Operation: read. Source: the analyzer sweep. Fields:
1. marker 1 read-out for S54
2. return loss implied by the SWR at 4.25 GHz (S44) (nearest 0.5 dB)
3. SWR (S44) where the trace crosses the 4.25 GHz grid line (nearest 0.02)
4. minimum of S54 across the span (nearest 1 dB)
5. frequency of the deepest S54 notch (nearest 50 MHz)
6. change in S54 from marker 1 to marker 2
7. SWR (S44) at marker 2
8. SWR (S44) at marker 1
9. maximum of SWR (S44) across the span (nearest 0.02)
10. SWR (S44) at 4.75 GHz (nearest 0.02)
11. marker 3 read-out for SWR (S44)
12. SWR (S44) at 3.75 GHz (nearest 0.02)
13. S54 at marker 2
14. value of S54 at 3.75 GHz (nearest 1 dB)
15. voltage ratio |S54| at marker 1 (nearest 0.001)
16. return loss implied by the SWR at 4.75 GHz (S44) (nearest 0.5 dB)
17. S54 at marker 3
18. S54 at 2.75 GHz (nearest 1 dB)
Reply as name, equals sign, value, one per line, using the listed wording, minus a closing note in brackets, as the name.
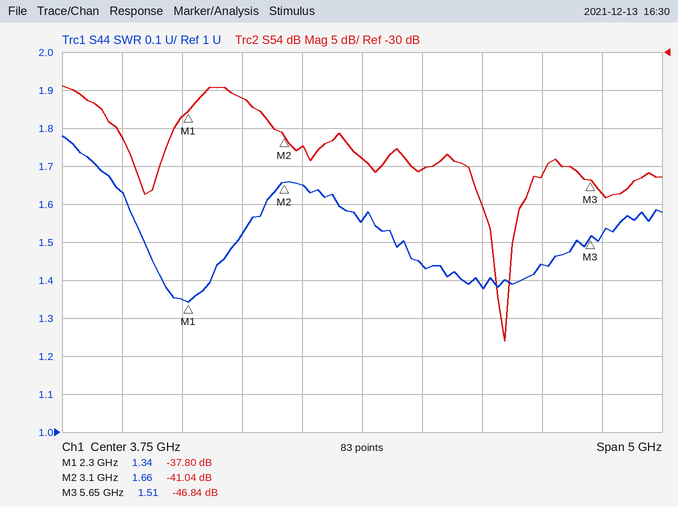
marker 1 read-out for S54 = -37.80 dB
return loss implied by the SWR at 4.25 GHz (S44) = 15.0 dB
SWR (S44) where the trace crosses the 4.25 GHz grid line = 1.44
minimum of S54 across the span = -68 dB
frequency of the deepest S54 notch = 4.95 GHz
change in S54 from marker 1 to marker 2 = -3.24 dB
SWR (S44) at marker 2 = 1.66
SWR (S44) at marker 1 = 1.34
maximum of SWR (S44) across the span = 1.78
SWR (S44) at 4.75 GHz = 1.38
marker 3 read-out for SWR = 1.51
SWR (S44) at 3.75 GHz = 1.56
S54 at marker 2 = -41.04 dB
value of S54 at 3.75 GHz = -44 dB
voltage ratio |S54| at marker 1 = 0.013
return loss implied by the SWR at 4.75 GHz (S44) = 16.0 dB
S54 at marker 3 = -46.84 dB
S54 at 2.75 GHz = -36 dB
